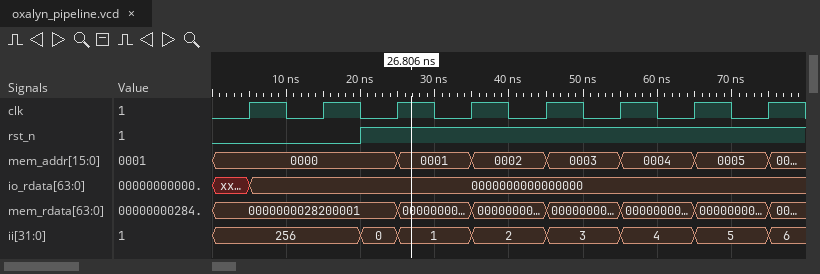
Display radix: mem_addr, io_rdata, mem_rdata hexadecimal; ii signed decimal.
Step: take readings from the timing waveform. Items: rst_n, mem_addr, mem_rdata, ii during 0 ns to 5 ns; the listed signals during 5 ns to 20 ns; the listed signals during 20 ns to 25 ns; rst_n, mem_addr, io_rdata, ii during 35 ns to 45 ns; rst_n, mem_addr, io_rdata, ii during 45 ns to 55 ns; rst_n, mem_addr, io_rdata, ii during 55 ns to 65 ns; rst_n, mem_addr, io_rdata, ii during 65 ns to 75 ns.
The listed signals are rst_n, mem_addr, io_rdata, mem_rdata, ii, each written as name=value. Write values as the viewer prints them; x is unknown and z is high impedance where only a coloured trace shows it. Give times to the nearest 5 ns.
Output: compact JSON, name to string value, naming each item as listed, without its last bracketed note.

{"rst_n, mem_addr, mem_rdata, ii during 0 ns to 5 ns": "rst_n=0, mem_addr=0000, mem_rdata=0000000028200001, ii=256", "the listed signals during 5 ns to 20 ns": "rst_n=0, mem_addr=0000, io_rdata=0000000000000000, mem_rdata=0000000028200001, ii=256", "the listed signals during 20 ns to 25 ns": "rst_n=1, mem_addr=0000, io_rdata=0000000000000000, mem_rdata=0000000028200001, ii=0", "rst_n, mem_addr, io_rdata, ii during 35 ns to 45 ns": "rst_n=1, mem_addr=0002, io_rdata=0000000000000000, ii=2", "rst_n, mem_addr, io_rdata, ii during 45 ns to 55 ns": "rst_n=1, mem_addr=0003, io_rdata=0000000000000000, ii=3", "rst_n, mem_addr, io_rdata, ii during 55 ns to 65 ns": "rst_n=1, mem_addr=0004, io_rdata=0000000000000000, ii=4", "rst_n, mem_addr, io_rdata, ii during 65 ns to 75 ns": "rst_n=1, mem_addr=0005, io_rdata=0000000000000000, ii=5"}
